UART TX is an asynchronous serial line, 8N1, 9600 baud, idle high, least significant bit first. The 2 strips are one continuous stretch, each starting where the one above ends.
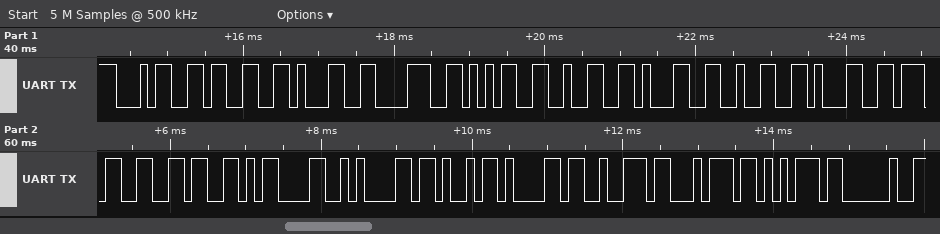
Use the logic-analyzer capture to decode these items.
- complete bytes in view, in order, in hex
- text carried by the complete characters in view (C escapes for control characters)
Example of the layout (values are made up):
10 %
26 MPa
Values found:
34 33 31 38 35 32 31 32 31 37 36 0D 0A 4B 61 72 74 75 20
"43185212176\r\nKartu "
